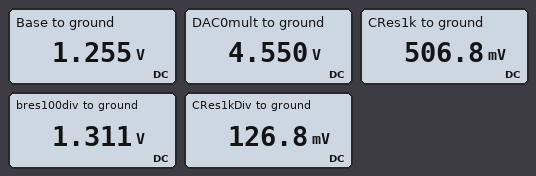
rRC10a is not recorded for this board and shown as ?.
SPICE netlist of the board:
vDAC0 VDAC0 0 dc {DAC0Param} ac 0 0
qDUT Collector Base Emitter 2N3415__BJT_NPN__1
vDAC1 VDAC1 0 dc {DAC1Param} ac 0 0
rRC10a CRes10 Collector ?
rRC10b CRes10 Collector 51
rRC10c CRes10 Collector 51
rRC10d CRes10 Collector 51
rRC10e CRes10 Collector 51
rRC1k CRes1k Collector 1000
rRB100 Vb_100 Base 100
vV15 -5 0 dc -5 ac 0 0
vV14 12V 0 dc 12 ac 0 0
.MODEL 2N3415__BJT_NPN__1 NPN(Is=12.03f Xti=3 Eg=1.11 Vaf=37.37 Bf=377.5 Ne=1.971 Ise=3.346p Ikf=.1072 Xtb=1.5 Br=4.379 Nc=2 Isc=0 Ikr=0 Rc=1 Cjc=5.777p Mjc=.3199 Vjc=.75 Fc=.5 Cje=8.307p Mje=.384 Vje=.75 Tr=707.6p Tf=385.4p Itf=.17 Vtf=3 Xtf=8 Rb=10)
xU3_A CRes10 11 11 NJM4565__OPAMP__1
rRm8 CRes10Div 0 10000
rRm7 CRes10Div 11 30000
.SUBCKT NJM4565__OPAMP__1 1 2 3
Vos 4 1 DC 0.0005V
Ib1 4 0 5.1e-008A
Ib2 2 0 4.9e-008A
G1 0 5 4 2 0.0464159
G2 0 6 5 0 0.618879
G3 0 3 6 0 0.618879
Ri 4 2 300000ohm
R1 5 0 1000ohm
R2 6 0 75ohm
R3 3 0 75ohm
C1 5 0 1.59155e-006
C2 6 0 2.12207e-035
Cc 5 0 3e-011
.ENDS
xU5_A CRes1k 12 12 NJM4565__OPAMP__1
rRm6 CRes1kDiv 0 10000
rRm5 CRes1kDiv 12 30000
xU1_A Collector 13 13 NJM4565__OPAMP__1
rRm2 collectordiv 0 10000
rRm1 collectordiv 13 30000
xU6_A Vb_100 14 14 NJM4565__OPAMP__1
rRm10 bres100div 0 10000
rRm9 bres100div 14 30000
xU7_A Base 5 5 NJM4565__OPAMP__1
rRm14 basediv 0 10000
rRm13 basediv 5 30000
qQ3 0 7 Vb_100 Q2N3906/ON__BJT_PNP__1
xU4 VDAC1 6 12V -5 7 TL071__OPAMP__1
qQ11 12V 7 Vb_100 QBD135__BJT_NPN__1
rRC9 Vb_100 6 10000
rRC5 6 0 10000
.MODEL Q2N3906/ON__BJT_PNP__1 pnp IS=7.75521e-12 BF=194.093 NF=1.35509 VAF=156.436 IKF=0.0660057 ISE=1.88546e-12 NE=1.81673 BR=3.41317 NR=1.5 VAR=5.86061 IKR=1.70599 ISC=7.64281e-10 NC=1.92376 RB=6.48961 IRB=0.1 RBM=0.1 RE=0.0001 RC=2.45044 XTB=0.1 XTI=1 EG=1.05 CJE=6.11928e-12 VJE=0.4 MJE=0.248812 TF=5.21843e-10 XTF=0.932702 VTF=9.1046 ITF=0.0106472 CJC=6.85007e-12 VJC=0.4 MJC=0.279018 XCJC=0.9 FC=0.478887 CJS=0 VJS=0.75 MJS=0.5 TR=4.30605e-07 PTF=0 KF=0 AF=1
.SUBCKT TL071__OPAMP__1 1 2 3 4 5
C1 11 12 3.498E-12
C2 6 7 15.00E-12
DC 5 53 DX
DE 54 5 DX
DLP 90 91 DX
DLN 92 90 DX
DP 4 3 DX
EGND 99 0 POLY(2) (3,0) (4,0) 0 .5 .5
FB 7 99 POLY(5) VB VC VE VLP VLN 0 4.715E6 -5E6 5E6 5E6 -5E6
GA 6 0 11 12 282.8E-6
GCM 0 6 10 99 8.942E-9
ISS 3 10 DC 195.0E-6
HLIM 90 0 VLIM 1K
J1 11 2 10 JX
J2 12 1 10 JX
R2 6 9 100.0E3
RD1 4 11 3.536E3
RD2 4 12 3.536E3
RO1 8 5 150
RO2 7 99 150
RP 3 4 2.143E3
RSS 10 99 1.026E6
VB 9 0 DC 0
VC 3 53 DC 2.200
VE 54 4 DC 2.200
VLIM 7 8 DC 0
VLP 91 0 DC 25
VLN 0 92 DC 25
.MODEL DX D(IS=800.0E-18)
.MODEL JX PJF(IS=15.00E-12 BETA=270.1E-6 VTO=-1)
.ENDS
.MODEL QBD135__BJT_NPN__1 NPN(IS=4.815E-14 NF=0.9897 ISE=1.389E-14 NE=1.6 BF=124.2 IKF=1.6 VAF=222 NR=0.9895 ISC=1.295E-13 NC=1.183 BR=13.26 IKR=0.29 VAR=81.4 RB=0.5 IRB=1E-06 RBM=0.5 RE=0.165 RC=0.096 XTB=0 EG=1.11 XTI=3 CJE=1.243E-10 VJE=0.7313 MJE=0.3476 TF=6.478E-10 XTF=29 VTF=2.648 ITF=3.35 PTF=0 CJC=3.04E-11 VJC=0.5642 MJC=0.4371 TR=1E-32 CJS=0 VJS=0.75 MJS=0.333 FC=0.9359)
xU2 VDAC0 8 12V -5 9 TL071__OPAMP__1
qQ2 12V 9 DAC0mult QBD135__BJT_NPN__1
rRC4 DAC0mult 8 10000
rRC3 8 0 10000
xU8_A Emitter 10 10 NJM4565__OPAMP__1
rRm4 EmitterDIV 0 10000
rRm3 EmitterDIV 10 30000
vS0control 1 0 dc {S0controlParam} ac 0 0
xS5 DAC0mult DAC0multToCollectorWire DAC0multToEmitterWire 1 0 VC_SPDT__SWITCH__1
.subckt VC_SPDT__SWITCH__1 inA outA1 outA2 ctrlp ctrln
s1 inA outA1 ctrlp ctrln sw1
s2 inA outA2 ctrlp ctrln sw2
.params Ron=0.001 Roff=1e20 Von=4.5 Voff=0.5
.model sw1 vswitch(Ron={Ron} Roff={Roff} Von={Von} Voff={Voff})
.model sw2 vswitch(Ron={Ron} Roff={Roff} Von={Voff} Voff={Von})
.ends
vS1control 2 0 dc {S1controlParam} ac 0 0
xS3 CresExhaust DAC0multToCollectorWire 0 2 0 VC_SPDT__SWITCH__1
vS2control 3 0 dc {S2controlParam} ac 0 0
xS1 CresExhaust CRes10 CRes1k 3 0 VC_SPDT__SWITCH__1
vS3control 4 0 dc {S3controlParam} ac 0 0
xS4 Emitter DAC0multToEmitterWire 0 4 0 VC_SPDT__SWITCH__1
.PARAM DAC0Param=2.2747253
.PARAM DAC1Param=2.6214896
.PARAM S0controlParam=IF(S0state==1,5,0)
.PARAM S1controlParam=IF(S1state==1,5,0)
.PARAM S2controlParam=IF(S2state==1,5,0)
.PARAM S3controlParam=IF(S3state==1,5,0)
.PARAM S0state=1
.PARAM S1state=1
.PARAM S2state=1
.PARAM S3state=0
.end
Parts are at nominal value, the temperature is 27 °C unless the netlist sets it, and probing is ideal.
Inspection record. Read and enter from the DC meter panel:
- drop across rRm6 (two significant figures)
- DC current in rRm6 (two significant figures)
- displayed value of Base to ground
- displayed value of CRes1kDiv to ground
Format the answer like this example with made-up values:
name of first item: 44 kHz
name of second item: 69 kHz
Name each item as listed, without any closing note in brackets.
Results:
drop across rRm6: 130 mV
DC current in rRm6: 13 µA
displayed value of Base to ground: 1.255 V
displayed value of CRes1kDiv to ground: 126.8 mV
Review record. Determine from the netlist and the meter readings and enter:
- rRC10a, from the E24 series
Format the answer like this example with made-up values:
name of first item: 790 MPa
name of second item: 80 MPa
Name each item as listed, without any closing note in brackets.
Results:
rRC10a, from the E24 series: 36 Ω
